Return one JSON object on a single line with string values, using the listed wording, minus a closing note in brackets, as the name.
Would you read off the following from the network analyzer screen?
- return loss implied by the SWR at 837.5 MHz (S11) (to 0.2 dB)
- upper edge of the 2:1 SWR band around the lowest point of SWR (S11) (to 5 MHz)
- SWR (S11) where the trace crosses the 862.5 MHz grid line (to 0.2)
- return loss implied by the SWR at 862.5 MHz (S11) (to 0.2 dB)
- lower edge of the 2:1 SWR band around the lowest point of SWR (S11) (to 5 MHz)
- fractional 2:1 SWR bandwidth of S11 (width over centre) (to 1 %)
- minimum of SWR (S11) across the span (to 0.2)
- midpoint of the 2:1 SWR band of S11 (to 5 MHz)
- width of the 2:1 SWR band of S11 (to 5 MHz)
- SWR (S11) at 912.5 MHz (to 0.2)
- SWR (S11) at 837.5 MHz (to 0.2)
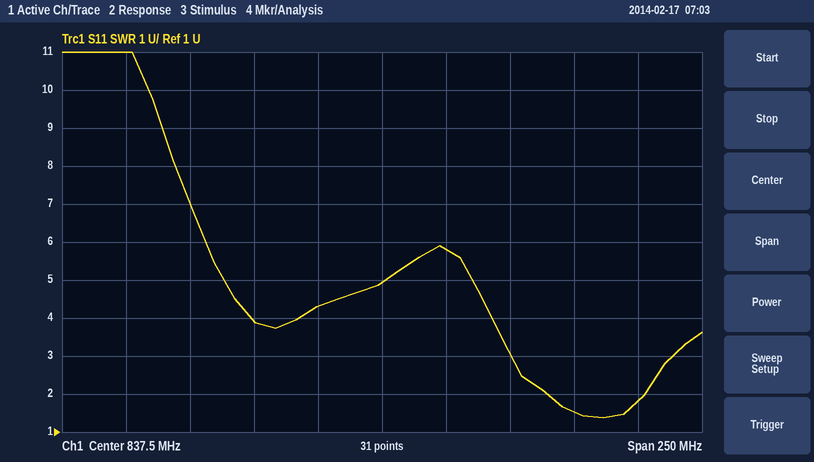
{"return loss implied by the SWR at 837.5 MHz (S11)": "3.6 dB", "upper edge of the 2:1 SWR band around the lowest point of SWR (S11)": "940 MHz", "SWR (S11) where the trace crosses the 862.5 MHz grid line": "5.8", "return loss implied by the SWR at 862.5 MHz (S11)": "3.0 dB", "lower edge of the 2:1 SWR band around the lowest point of SWR (S11)": "900 MHz", "fractional 2:1 SWR bandwidth of S11 (width over centre)": "4 %", "minimum of SWR (S11) across the span": "1.4", "midpoint of the 2:1 SWR band of S11": "920 MHz", "width of the 2:1 SWR band of S11": "40 MHz", "SWR (S11) at 912.5 MHz": "1.6", "SWR (S11) at 837.5 MHz": "5.0"}
